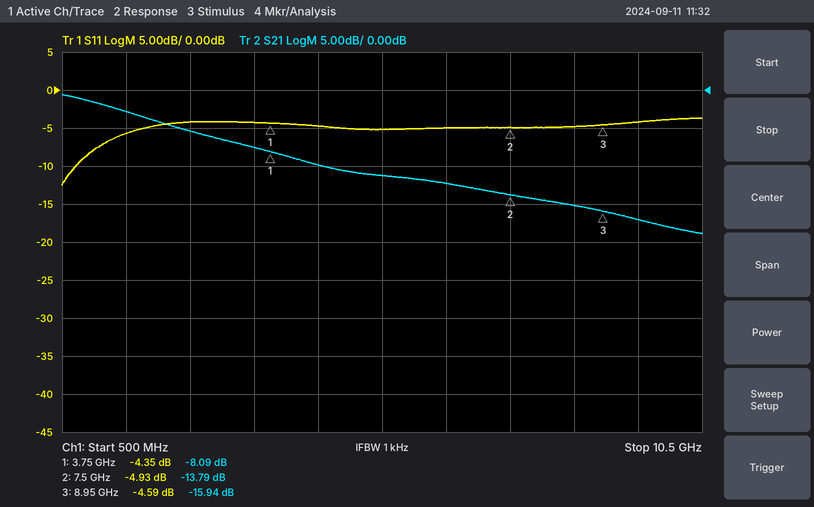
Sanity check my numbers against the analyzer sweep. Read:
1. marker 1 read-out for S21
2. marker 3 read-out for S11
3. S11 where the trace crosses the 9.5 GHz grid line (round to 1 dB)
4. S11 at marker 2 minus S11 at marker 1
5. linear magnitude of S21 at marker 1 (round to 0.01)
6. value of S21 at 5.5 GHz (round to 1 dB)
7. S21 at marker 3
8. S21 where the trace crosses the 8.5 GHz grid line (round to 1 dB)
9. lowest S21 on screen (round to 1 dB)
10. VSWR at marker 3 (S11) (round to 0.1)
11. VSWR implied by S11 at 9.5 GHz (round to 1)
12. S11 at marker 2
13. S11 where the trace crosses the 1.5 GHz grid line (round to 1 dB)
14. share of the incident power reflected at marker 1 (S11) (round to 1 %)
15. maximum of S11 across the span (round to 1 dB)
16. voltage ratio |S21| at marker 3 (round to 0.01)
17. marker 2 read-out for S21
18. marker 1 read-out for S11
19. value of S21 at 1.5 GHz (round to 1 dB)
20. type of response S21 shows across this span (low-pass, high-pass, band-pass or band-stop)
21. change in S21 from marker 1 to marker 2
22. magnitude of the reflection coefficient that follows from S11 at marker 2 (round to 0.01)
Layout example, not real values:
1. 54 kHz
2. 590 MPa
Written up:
1. -8.09 dB
2. -4.59 dB
3. -4 dB
4. -0.58 dB
5. 0.39
6. -11 dB
7. -15.94 dB
8. -15 dB
9. -19 dB
10. 3.9
11. 4
12. -4.93 dB
13. -6 dB
14. 37 %
15. -4 dB
16. 0.16
17. -13.79 dB
18. -4.35 dB
19. -3 dB
20. low-pass
21. -5.70 dB
22. 0.57
